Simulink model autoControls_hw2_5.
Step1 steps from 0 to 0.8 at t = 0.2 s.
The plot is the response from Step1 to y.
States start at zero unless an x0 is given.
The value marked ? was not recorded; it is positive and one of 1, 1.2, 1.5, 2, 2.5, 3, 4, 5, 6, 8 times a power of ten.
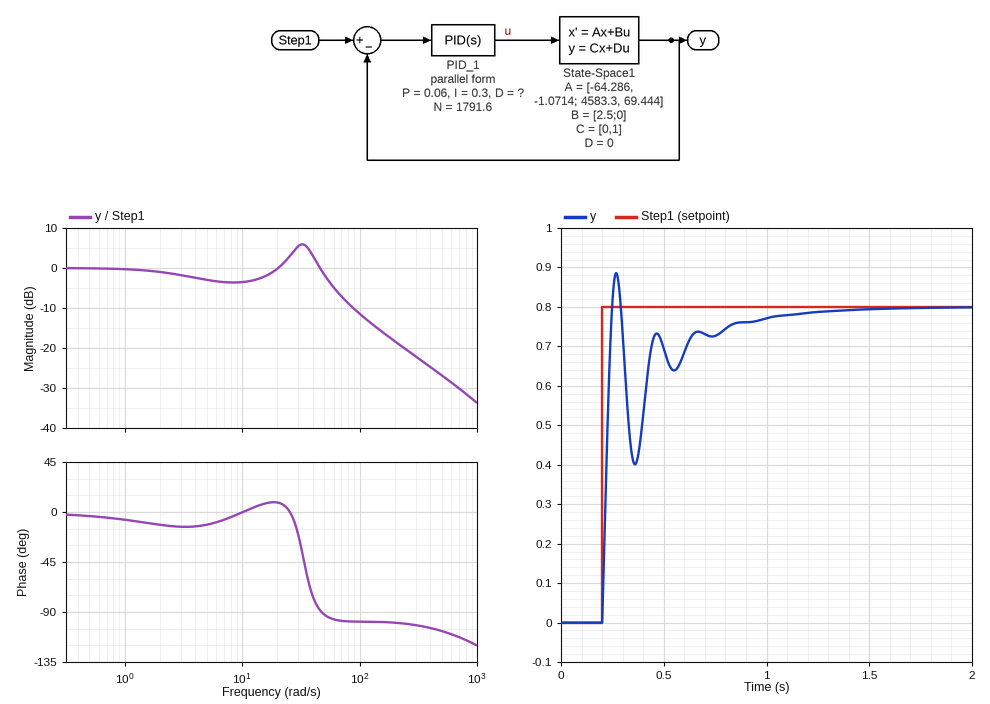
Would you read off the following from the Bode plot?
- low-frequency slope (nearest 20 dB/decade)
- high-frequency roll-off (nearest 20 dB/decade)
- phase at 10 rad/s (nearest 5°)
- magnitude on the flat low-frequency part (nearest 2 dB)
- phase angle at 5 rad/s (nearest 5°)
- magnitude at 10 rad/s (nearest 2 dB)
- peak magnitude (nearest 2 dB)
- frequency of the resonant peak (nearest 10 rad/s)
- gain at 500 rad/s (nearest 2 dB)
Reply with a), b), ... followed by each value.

a) 0 dB/decade
b) -20 dB/decade
c) 0°
d) 0 dB
e) -10°
f) -4 dB
g) 6 dB
h) 30 rad/s
i) -26 dB
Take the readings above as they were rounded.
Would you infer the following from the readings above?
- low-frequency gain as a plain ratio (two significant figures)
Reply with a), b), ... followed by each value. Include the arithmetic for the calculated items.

a) 10^(0 / 20) = 1.0
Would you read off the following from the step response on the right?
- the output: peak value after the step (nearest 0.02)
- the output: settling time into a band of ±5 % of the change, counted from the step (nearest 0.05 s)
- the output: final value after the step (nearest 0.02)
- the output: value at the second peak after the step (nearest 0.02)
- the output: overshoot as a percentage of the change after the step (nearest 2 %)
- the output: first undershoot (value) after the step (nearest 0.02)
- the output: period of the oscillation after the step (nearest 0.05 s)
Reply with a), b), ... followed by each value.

a) 0.88
b) 0.65 s
c) 0.80
d) 0.74
e) 10 %
f) 0.40
g) 0.20 s
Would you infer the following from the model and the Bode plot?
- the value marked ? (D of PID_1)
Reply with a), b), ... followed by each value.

a) 0.002
